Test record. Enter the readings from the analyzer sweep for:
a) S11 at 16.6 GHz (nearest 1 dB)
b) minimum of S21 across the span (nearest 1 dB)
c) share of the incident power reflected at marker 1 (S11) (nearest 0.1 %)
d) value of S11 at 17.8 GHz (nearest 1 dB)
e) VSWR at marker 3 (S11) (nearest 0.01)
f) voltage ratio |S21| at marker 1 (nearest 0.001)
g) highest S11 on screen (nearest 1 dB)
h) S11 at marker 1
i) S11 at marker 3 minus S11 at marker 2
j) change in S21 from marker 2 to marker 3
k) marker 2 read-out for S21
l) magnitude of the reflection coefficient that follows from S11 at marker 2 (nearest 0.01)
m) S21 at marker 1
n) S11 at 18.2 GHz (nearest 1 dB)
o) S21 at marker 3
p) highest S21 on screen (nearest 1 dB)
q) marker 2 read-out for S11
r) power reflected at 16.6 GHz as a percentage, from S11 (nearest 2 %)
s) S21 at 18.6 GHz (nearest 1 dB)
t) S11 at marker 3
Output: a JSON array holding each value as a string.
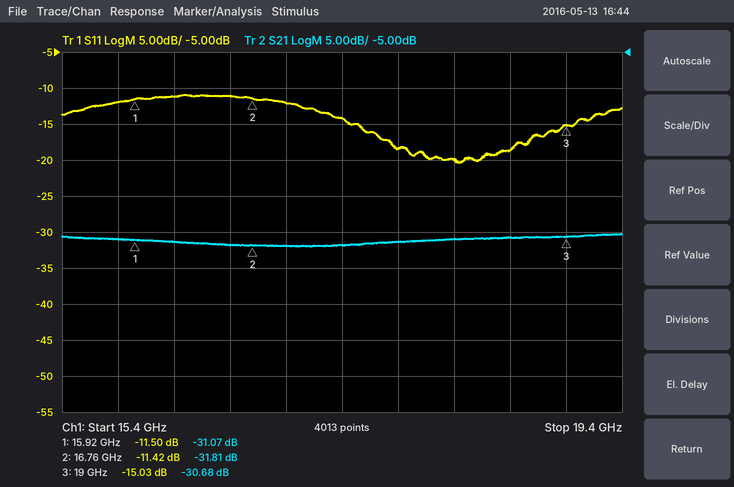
["-11 dB", "-32 dB", "7.1 %", "-18 dB", "1.43", "0.028", "-11 dB", "-11.50 dB", "-3.61 dB", "1.13 dB", "-31.81 dB", "0.27", "-31.07 dB", "-20 dB", "-30.68 dB", "-30 dB", "-11.42 dB", "8 %", "-31 dB", "-15.03 dB"]
